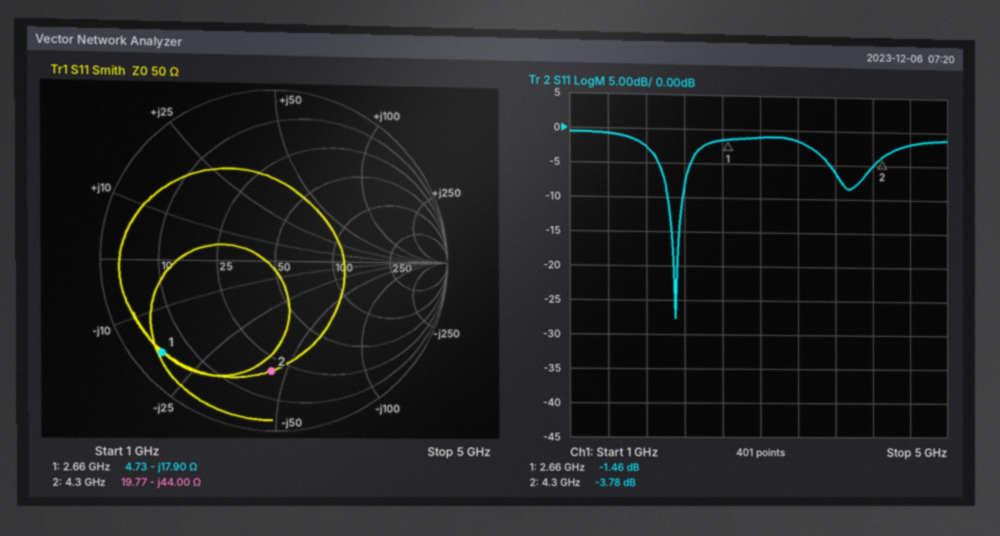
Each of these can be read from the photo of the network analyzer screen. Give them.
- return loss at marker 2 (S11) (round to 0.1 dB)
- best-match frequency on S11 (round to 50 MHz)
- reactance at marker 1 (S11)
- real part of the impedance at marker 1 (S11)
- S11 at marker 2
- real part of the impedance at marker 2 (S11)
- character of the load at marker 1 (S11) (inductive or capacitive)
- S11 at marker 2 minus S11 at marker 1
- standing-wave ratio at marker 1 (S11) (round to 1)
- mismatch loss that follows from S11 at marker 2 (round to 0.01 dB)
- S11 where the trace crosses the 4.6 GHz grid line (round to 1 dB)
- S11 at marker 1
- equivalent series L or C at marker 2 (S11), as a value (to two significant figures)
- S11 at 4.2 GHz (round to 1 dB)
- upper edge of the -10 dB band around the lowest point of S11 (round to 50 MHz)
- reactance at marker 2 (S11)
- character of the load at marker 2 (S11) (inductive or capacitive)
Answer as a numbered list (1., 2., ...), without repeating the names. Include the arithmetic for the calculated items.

1. 3.8 dB
2. 2.10 GHz
3. -17.90 Ω
4. 4.73 Ω
5. -3.78 dB
6. 19.77 Ω
7. capacitive
8. -3.78 − (-1.46) = -2.32 dB
9. 12
10. −10 log10(1 − 10^(-3.78/10)) ≈ 2.36 dB
11. -2 dB
12. -1.46 dB
13. C = 1/(2π × 4.3 GHz × 44 Ω) ≈ 841 fF, so 840 fF to two significant figures
14. -5 dB
15. 2.20 GHz
16. -44.00 Ω
17. capacitive
